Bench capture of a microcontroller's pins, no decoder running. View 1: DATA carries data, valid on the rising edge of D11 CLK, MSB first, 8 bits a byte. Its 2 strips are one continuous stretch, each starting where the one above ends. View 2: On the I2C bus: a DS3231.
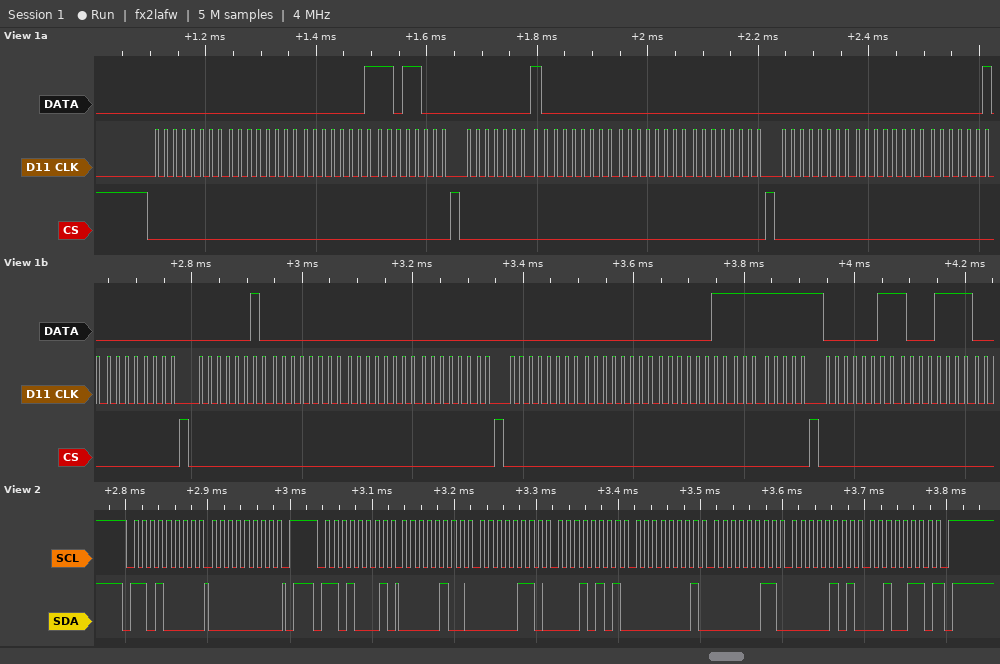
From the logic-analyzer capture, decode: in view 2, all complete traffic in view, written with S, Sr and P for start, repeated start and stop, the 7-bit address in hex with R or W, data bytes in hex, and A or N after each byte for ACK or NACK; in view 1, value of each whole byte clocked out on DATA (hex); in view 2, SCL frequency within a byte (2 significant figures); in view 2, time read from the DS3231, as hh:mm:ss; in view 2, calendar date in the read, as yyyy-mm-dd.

S 68W A 00 A P S 68R A 04 A 06 A 15 A 01 A 03 A 05 A 26 N P
00 00 01 D8 01 00 00 00 00 00 02 00 02 00 00 00 00 00 03 FF 03 8F
100 kHz
15:06:04
2026-05-03
